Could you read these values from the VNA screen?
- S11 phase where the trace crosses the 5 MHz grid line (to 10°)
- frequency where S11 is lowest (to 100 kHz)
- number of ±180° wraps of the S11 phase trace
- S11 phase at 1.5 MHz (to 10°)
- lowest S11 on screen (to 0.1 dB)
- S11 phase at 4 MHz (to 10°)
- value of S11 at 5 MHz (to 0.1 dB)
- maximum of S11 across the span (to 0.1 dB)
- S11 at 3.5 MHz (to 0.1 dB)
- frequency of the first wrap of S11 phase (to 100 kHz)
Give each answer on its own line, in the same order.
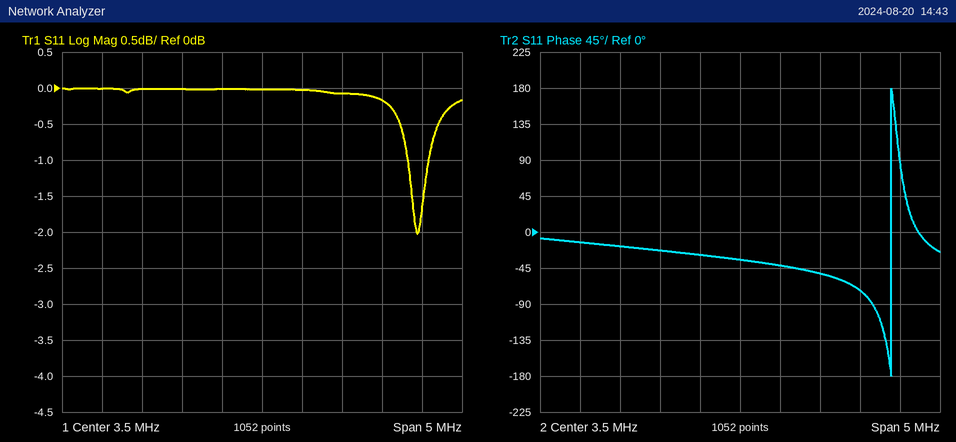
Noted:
-70°
5.4 MHz
1
-10°
-2.0 dB
-40°
-0.2 dB
0.0 dB
0.0 dB
5.4 MHz
